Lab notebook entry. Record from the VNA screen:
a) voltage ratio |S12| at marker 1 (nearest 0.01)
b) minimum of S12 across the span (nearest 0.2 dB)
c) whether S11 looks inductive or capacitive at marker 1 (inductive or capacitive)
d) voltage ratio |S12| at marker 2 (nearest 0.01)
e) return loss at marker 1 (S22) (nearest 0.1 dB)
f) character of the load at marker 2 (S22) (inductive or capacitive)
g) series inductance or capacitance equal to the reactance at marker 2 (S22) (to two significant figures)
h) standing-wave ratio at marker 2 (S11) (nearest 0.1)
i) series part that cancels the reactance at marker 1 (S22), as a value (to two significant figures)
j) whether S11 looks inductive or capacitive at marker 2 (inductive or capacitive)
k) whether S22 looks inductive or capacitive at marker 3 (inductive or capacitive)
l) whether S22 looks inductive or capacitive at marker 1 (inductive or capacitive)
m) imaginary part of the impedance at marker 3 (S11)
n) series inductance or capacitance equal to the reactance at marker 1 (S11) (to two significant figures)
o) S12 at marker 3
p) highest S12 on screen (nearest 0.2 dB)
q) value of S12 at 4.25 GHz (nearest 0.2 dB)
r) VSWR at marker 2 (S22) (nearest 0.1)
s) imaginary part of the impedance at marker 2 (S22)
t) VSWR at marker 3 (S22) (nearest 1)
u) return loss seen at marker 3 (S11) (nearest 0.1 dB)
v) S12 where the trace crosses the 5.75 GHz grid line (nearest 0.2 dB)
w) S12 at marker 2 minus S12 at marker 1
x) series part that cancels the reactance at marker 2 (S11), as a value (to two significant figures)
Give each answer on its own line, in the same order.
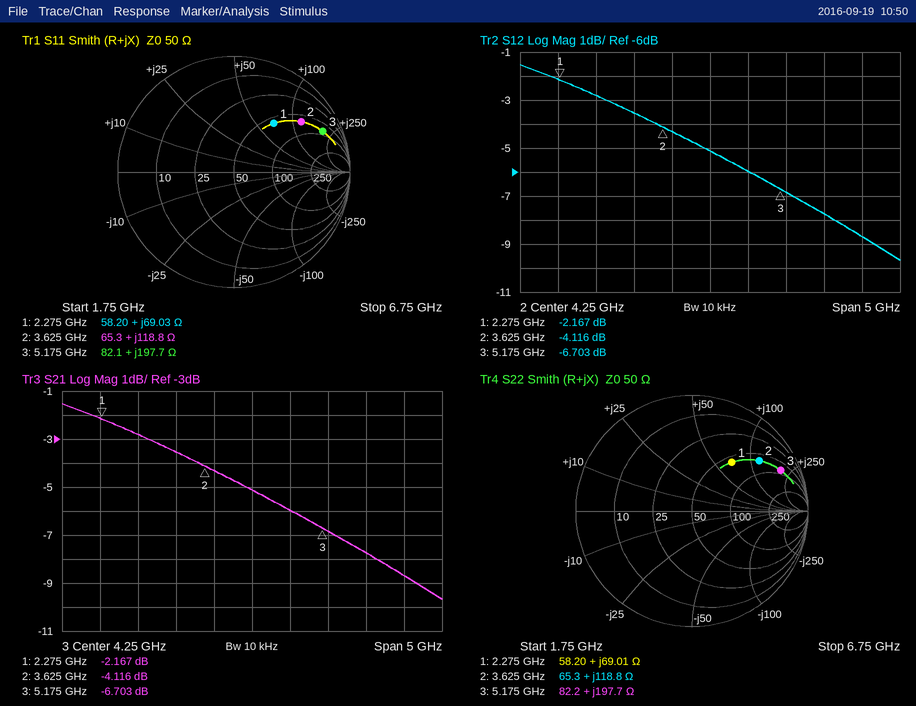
0.78
-9.6 dB
inductive
0.62
5.3 dB
inductive
5.2 nH
6.2
1.0 pF
inductive
inductive
inductive
+197.7 Ω
4.8 nH
-6.703 dB
-1.6 dB
-5.2 dB
6.2
+118.8 Ω
12
1.5 dB
-7.8 dB
-1.949 dB
370 fF
